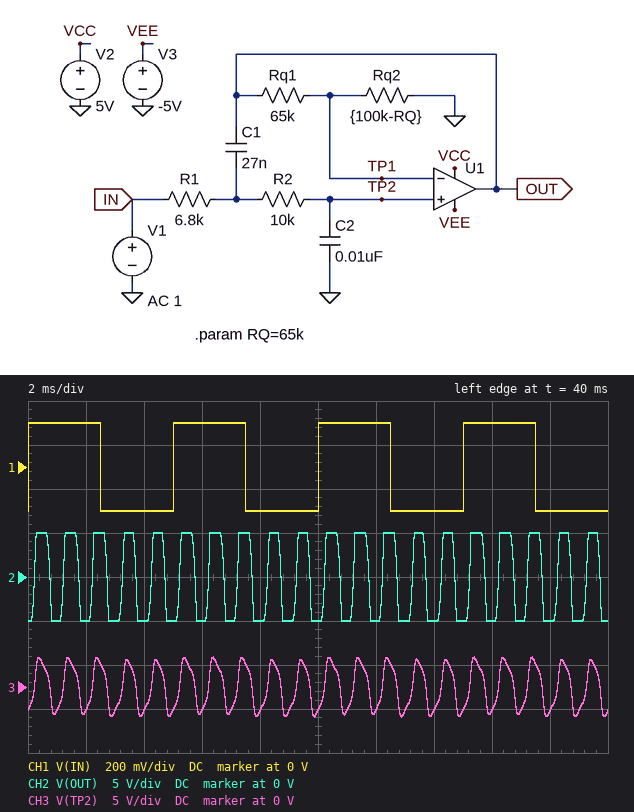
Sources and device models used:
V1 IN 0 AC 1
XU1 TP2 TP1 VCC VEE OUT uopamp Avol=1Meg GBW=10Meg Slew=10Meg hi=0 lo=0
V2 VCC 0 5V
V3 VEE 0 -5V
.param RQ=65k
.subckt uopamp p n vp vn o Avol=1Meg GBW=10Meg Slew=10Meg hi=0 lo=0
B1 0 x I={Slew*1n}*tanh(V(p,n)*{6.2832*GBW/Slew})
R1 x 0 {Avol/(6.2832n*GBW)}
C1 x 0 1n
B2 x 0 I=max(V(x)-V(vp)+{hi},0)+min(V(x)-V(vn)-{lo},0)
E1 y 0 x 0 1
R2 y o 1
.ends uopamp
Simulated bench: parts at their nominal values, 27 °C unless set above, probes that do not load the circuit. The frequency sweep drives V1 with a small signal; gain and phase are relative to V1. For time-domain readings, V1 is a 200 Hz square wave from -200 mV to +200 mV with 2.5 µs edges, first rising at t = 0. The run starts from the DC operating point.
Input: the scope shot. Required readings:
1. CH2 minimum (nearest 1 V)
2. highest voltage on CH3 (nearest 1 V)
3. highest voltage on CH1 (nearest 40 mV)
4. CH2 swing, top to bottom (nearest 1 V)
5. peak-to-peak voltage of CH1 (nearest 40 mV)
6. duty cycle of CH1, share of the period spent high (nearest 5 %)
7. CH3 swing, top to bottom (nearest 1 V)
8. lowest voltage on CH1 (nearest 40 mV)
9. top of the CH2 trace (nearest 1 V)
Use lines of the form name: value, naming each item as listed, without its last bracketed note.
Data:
CH2 minimum: -5 V
highest voltage on CH3: 3 V
highest voltage on CH1: 200 mV
CH2 swing, top to bottom: 10 V
peak-to-peak voltage of CH1: 400 mV
duty cycle of CH1, share of the period spent high: 50 %
CH3 swing, top to bottom: 7 V
lowest voltage on CH1: -200 mV
top of the CH2 trace: 5 V
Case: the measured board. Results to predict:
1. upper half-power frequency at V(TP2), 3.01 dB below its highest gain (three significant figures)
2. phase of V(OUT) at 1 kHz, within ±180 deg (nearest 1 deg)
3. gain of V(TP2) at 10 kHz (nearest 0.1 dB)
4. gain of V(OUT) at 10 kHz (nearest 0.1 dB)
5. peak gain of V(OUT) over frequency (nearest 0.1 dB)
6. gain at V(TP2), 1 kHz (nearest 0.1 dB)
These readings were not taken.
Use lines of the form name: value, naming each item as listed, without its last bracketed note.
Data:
upper half-power frequency at V(TP2), 3.01 dB below its highest gain: 1.27 kHz
phase of V(OUT) at 1 kHz, within ±180 deg: 76 deg
gain of V(TP2) at 10 kHz: -37.2 dB
gain of V(OUT) at 10 kHz: -28.1 dB
peak gain of V(OUT) over frequency: 9.3 dB
gain at V(TP2), 1 kHz: -1.0 dB
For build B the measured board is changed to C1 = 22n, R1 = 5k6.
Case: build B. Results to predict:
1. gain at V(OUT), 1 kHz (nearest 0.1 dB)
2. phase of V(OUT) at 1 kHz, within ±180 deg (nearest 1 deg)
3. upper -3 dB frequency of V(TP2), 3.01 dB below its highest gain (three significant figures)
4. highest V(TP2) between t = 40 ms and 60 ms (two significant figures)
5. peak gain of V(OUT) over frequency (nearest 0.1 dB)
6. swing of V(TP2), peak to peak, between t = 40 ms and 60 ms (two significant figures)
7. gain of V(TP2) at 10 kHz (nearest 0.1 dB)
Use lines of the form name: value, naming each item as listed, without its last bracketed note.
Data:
gain at V(OUT), 1 kHz: 12.4 dB
phase of V(OUT) at 1 kHz, within ±180 deg: 42 deg
upper -3 dB frequency of V(TP2), 3.01 dB below its highest gain: 1.70 kHz
highest V(TP2) between t = 40 ms and 60 ms: 2.7 V
peak gain of V(OUT) over frequency: 13.3 dB
swing of V(TP2), peak to peak, between t = 40 ms and 60 ms: 5.5 V
gain of V(TP2) at 10 kHz: -33.6 dB
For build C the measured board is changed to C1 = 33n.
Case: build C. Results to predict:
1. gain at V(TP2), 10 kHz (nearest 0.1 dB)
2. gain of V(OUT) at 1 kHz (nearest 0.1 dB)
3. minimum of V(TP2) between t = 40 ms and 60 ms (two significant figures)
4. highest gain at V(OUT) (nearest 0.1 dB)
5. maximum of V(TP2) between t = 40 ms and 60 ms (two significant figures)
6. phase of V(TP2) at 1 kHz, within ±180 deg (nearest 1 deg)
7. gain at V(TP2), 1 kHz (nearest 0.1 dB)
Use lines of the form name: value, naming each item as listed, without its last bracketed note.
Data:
gain at V(TP2), 10 kHz: -39.0 dB
gain of V(OUT) at 1 kHz: 5.2 dB
minimum of V(TP2) between t = 40 ms and 60 ms: -3.7 V
highest gain at V(OUT): 9.1 dB
maximum of V(TP2) between t = 40 ms and 60 ms: 3.7 V
phase of V(TP2) at 1 kHz, within ±180 deg: 86 deg
gain at V(TP2), 1 kHz: -3.9 dB
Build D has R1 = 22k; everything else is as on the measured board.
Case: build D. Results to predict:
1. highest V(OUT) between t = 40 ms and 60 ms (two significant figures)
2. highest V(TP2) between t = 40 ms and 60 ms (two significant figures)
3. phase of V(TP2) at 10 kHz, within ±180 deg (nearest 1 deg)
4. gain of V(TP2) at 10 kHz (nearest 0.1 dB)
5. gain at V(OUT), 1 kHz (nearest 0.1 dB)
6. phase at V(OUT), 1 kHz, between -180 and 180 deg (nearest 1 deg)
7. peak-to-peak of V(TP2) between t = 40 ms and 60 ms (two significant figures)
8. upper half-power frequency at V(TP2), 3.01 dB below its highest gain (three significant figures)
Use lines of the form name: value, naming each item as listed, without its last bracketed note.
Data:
highest V(OUT) between t = 40 ms and 60 ms: 5.0 V
highest V(TP2) between t = 40 ms and 60 ms: 4.5 V
phase of V(TP2) at 10 kHz, within ±180 deg: 168 deg
gain of V(TP2) at 10 kHz: -47.6 dB
gain at V(OUT), 1 kHz: -5.0 dB
phase at V(OUT), 1 kHz, between -180 and 180 deg: 105 deg
peak-to-peak of V(TP2) between t = 40 ms and 60 ms: 8.9 V
upper half-power frequency at V(TP2), 3.01 dB below its highest gain: 225 Hz
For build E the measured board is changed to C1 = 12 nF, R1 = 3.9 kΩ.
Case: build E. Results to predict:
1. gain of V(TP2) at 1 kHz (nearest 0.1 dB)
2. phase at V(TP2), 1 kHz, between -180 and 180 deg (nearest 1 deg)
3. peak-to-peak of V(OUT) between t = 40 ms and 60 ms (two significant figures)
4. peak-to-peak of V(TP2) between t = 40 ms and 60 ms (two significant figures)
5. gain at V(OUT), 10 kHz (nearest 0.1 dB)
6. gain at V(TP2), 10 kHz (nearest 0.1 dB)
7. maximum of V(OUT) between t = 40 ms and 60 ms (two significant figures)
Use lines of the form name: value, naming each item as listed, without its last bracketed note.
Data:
gain of V(TP2) at 1 kHz: 1.1 dB
phase at V(TP2), 1 kHz, between -180 and 180 deg: -22 deg
peak-to-peak of V(OUT) between t = 40 ms and 60 ms: 1.8 V
peak-to-peak of V(TP2) between t = 40 ms and 60 ms: 620 mV
gain at V(OUT), 10 kHz: -15.9 dB
gain at V(TP2), 10 kHz: -25.0 dB
maximum of V(OUT) between t = 40 ms and 60 ms: 890 mV
